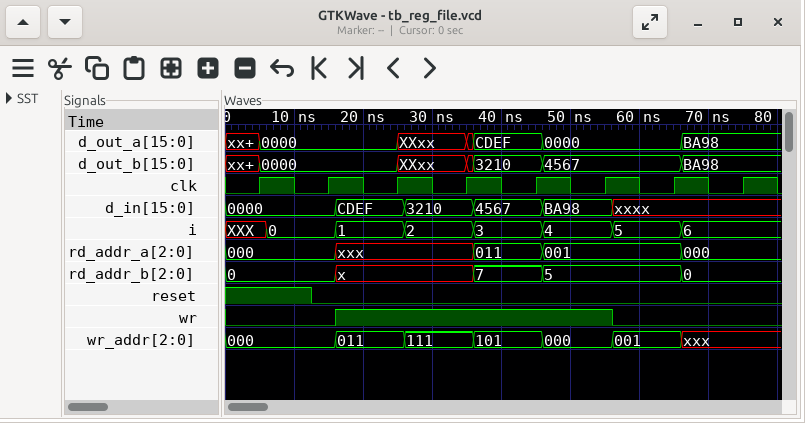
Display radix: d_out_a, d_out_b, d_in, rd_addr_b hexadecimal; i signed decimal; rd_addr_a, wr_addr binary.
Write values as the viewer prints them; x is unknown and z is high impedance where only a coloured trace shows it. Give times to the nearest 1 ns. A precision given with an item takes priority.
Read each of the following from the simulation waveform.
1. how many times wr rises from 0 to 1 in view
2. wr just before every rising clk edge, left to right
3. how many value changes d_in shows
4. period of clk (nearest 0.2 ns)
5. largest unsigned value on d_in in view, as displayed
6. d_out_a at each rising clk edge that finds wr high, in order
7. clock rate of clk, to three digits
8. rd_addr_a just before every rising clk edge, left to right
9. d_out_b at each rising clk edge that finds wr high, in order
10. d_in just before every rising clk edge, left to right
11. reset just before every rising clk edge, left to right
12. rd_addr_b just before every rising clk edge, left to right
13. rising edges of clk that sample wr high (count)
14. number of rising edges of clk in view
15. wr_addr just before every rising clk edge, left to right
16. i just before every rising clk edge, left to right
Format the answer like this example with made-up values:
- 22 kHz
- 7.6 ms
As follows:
- 1
- 0 0 1 1 1 1 0 0
- 5
- 10 ns
- CDEF
- 0000, XXxx, CDEF, 0000
- 100 MHz
- 000, 000, xxx, xxx, 011, 001, 001, 000
- 0000, XXxx, 3210, 4567
- 0000, 0000, CDEF, 3210, 4567, BA98, xxxx, xxxx
- 1 0 0 0 0 0 0 0
- 0, 0, x, x, 7, 5, 5, 0
- 4
- 8
- 000, 000, 011, 111, 101, 000, 001, xxx
- XXX, 0, 1, 2, 3, 4, 5, 6
